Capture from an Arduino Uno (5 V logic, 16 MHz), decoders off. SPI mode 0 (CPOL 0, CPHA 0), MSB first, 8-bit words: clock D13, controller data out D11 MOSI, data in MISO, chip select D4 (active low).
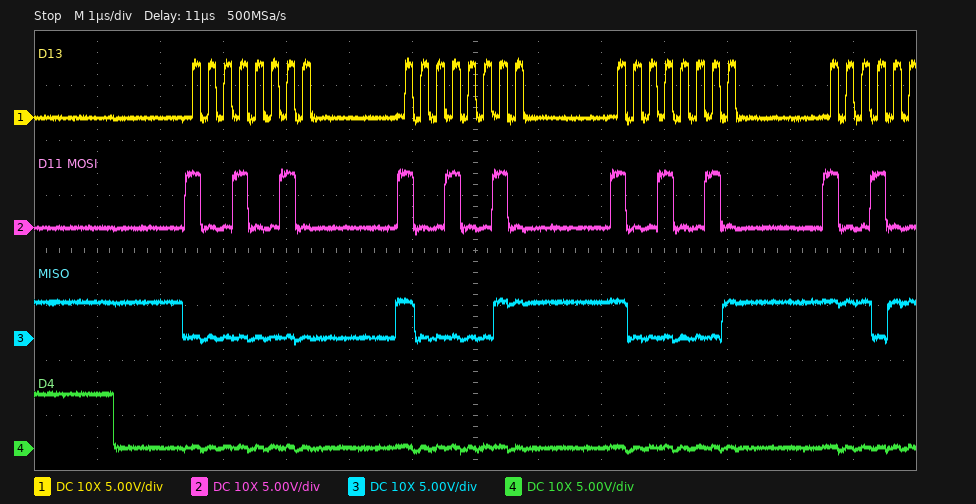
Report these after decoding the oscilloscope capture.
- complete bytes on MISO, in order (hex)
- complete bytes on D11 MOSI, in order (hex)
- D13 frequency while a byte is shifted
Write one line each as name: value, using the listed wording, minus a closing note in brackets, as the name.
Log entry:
complete bytes on MISO, in order: 00 83 81
complete bytes on D11 MOSI, in order: 92 92 92
D13 frequency while a byte is shifted: 4 MHz
